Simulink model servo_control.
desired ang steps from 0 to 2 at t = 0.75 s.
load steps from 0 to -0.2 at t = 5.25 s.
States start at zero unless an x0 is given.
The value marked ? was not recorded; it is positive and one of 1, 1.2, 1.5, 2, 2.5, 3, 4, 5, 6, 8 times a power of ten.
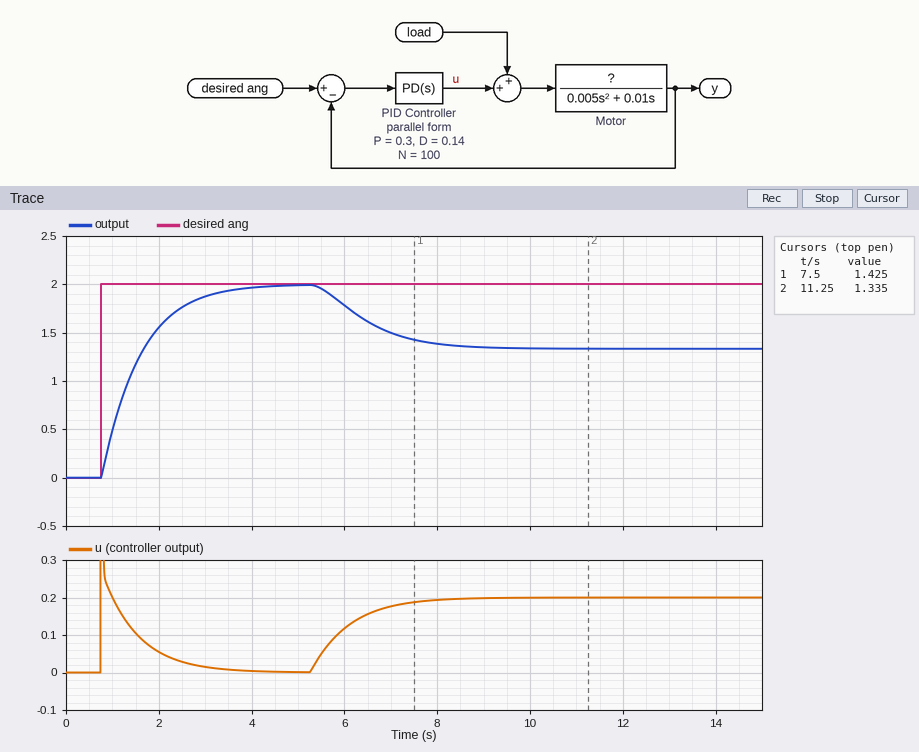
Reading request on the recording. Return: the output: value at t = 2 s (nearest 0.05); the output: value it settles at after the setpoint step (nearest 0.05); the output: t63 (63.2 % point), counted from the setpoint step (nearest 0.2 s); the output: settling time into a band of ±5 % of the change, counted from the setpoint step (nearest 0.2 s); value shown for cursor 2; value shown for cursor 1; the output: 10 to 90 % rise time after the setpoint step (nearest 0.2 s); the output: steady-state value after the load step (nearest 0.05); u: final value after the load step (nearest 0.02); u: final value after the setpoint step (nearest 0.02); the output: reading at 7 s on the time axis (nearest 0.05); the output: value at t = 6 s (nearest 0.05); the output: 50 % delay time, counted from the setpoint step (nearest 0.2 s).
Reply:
1.55
2.00
0.8 s
2.4 s
1.335
1.425
1.8 s
1.35
0.20
0.00
1.50
1.80
0.6 s
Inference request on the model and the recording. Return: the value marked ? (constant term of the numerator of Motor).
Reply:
0.04
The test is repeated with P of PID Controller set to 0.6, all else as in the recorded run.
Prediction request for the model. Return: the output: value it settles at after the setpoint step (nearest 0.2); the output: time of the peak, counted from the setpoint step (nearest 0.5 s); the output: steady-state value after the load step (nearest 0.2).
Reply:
2.0
1.5 s
1.6
